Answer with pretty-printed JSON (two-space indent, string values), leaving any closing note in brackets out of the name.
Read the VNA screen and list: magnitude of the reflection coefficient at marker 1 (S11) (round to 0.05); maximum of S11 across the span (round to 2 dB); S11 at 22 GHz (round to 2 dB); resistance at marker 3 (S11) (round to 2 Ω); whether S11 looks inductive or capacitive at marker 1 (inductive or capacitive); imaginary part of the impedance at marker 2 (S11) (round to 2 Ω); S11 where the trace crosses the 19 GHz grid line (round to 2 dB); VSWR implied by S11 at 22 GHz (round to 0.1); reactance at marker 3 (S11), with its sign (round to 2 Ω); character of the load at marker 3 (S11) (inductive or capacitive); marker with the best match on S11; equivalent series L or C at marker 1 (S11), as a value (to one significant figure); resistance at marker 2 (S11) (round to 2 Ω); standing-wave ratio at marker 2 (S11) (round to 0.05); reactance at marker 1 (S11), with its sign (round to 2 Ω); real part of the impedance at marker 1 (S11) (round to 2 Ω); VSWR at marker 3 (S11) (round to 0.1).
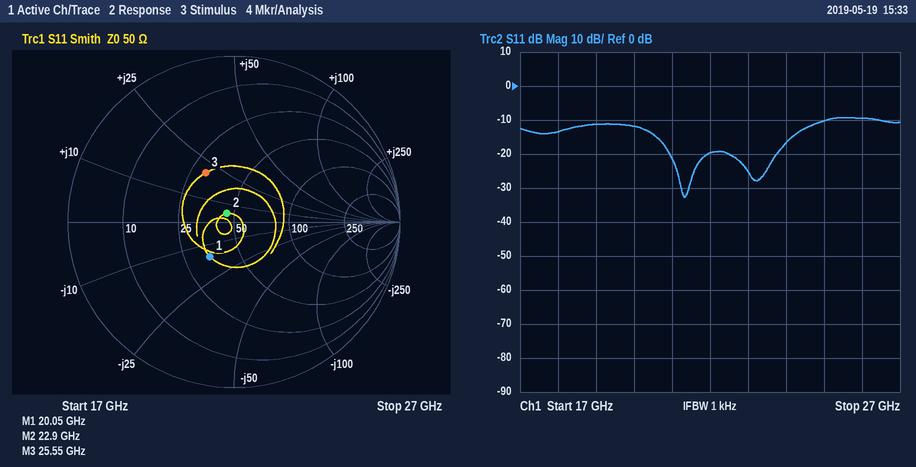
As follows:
{
  "magnitude of the reflection coefficient at marker 1 (S11)": "0.25",
  "maximum of S11 across the span": "-10 dB",
  "S11 at 22 GHz": "-20 dB",
  "resistance at marker 3 (S11)": "30 Ω",
  "whether S11 looks inductive or capacitive at marker 1": "capacitive",
  "imaginary part of the impedance at marker 2 (S11)": "+4 Ω",
  "S11 where the trace crosses the 19 GHz grid line": "-12 dB",
  "VSWR implied by S11 at 22 GHz": "1.2",
  "reactance at marker 3 (S11), with its sign": "+20 Ω",
  "character of the load at marker 3 (S11)": "inductive",
  "marker with the best match on S11": "marker 2",
  "equivalent series L or C at marker 1 (S11), as a value": "500 fF",
  "resistance at marker 2 (S11)": "46 Ω",
  "standing-wave ratio at marker 2 (S11)": "1.15",
  "reactance at marker 1 (S11), with its sign": "-16 Ω",
  "real part of the impedance at marker 1 (S11)": "34 Ω",
  "VSWR at marker 3 (S11)": "2.0"
}
